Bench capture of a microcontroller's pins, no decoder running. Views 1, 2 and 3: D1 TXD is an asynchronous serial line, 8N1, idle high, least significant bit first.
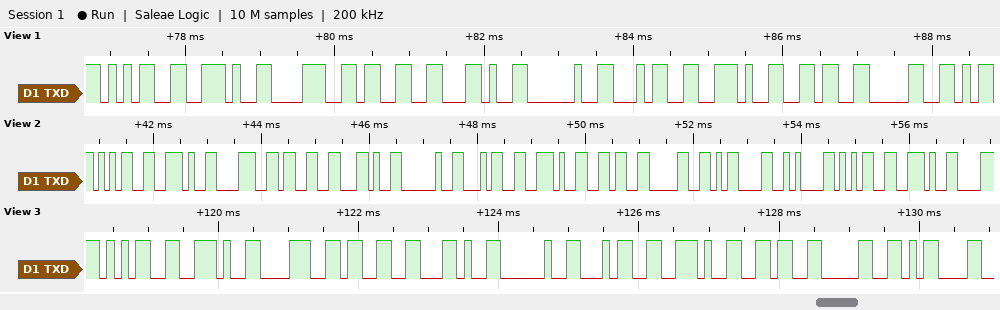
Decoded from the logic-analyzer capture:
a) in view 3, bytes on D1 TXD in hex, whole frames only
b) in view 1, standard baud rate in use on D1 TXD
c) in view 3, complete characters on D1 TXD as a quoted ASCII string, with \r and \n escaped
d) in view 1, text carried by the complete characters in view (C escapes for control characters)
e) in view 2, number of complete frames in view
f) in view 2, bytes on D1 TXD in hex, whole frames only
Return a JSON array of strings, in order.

["35 2E 38 33 2C 20 34 2E 36 30 0D", "9600 baud", "\"5.83, 4.60\\r\"", "\"5.83, 4.60\"", "14", "35 2E 38 33 2C 20 34 2E 36 30 0D 0A 35 2E"]
